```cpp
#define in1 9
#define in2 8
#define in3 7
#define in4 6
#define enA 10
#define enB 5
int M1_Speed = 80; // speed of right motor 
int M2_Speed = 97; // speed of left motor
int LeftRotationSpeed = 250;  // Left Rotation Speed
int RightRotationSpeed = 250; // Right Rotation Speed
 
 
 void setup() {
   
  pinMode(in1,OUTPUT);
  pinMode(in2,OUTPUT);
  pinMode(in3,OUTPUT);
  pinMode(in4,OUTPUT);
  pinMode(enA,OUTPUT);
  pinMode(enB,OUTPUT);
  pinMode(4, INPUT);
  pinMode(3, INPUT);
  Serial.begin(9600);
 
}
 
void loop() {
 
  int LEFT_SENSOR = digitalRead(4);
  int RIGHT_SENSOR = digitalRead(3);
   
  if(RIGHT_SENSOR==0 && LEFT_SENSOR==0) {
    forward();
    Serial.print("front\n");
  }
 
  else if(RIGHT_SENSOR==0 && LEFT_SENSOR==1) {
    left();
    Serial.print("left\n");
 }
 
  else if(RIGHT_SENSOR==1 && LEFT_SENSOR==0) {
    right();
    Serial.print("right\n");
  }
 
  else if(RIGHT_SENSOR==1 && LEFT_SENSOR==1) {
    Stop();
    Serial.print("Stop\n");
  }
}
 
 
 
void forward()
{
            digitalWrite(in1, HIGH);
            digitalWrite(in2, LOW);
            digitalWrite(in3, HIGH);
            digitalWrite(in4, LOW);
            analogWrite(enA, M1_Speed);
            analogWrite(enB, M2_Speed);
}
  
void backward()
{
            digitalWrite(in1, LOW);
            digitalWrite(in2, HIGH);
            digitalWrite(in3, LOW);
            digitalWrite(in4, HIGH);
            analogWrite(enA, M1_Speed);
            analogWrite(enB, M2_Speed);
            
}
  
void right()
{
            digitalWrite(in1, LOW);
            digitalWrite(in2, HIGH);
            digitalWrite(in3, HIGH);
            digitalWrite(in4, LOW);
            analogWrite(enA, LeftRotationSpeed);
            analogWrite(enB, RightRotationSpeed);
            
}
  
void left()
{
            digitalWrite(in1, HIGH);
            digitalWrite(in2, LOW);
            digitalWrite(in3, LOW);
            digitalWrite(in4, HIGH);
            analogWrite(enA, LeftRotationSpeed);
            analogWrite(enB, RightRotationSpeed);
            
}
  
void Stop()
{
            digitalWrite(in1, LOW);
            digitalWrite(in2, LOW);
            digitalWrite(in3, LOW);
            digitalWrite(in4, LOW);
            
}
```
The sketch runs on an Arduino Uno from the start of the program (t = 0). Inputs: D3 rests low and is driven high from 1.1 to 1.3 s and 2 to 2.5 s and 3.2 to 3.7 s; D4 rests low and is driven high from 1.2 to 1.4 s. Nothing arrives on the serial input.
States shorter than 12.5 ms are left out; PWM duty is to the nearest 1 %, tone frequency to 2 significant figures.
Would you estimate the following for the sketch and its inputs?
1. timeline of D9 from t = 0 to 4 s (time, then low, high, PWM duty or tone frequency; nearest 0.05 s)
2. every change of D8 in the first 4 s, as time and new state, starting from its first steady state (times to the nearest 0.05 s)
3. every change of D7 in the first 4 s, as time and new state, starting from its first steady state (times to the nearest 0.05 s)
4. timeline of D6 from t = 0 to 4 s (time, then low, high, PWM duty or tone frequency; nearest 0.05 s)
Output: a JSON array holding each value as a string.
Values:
["0 s high; 1.1 s low; 1.3 s high; 2 s low; 2.5 s high; 3.2 s low; 3.7 s high", "0 s low; 1.1 s high; 1.2 s low; 2 s high; 2.5 s low; 3.2 s high; 3.7 s low", "0 s high; 1.2 s low; 1.4 s high", "0 s low; 1.3 s high; 1.4 s low"]
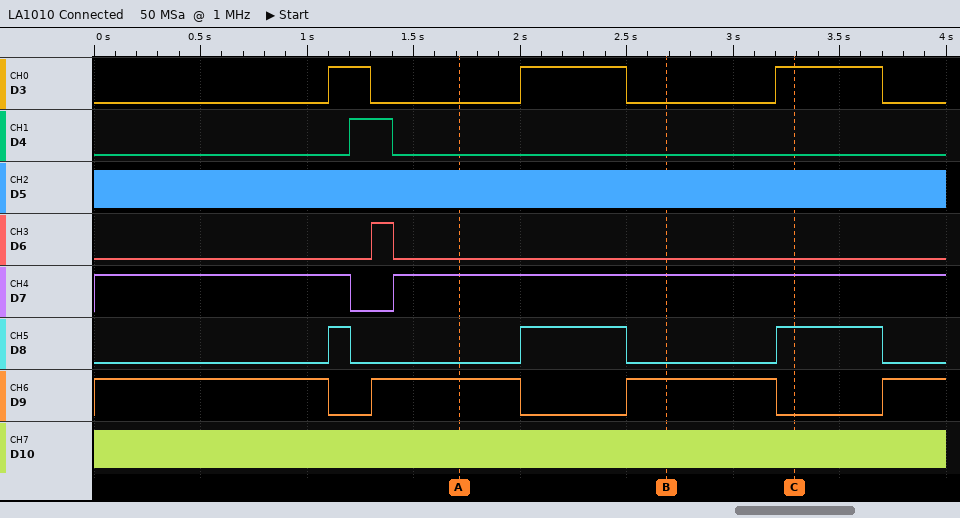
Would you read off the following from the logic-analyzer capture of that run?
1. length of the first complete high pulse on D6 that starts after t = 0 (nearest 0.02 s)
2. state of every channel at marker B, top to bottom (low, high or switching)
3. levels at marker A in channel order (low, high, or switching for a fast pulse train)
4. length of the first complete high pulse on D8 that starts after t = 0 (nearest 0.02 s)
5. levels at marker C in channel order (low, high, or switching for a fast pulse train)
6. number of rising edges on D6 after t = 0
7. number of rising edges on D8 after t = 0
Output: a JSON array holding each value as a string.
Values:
["0.10 s", "D3 low, D4 low, D5 switching, D6 low, D7 high, D8 low, D9 high, D10 switching", "D3 low, D4 low, D5 switching, D6 low, D7 high, D8 low, D9 high, D10 switching", "0.10 s", "D3 high, D4 low, D5 switching, D6 low, D7 high, D8 high, D9 low, D10 switching", "1", "3"]
